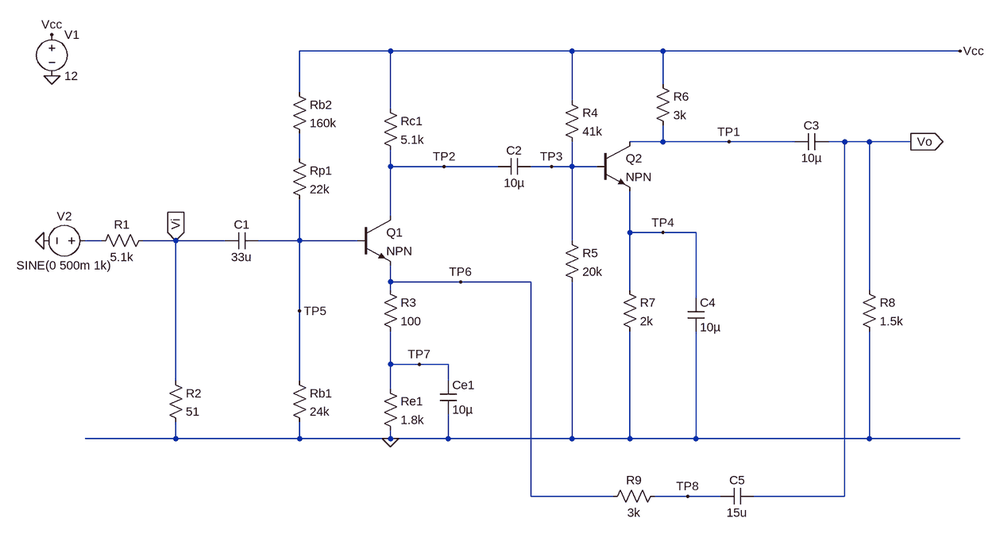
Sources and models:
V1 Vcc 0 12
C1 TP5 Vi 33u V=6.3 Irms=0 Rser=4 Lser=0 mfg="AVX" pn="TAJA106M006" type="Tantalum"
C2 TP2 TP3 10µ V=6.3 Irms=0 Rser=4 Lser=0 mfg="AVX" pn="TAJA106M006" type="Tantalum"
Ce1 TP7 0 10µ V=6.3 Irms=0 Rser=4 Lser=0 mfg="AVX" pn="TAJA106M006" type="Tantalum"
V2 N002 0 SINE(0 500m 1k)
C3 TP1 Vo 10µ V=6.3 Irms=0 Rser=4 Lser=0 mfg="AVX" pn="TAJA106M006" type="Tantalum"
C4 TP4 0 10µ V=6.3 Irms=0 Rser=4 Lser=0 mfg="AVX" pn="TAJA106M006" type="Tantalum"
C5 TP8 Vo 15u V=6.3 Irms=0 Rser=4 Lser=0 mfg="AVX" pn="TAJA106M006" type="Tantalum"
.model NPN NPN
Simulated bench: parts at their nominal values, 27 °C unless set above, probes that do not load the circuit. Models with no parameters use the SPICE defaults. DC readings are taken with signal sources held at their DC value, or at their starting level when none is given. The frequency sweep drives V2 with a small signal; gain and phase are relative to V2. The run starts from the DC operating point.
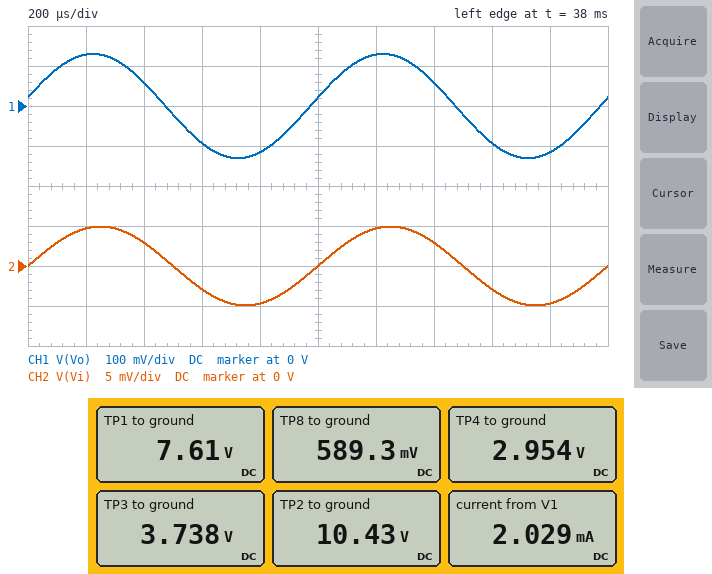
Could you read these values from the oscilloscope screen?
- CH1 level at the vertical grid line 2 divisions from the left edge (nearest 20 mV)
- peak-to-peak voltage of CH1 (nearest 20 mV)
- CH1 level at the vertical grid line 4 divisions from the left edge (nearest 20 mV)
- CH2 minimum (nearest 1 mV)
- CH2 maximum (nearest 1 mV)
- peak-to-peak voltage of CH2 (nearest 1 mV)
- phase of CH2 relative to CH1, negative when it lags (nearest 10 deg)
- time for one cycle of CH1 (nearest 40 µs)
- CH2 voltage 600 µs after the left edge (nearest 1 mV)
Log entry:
60 mV
260 mV
-120 mV
-5 mV
5 mV
10 mV
-10 deg
1.00 ms
-3 mV
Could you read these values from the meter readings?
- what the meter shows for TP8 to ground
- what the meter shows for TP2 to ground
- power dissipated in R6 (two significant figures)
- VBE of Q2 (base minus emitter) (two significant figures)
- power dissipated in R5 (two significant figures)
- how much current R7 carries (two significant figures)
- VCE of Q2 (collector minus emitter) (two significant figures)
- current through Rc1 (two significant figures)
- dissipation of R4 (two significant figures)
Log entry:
589.3 mV
10.43 V
6.4 mW
780 mV
700 µW
1.5 mA
4.7 V
310 µA
1.7 mW
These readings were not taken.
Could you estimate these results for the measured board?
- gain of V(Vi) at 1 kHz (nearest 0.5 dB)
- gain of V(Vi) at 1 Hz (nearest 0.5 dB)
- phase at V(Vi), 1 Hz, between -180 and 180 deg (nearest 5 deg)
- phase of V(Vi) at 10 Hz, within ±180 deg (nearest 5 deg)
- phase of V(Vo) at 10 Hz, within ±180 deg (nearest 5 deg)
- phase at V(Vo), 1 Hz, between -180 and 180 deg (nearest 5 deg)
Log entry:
-40.0 dB
-40.0 dB
0 deg
0 deg
70 deg
120 deg
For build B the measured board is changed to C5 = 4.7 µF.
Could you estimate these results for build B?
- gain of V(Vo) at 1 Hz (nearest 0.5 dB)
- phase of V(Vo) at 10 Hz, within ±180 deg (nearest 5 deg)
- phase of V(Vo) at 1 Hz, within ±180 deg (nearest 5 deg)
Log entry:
-54.0 dB
80 deg
135 deg
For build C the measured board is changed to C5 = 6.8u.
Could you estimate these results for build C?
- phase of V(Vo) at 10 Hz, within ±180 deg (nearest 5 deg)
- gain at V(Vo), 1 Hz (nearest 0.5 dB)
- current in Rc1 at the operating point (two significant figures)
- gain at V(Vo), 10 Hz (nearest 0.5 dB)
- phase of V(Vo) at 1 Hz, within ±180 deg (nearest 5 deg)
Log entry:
75 deg
-53.5 dB
310 µA
-34.0 dB
130 deg
